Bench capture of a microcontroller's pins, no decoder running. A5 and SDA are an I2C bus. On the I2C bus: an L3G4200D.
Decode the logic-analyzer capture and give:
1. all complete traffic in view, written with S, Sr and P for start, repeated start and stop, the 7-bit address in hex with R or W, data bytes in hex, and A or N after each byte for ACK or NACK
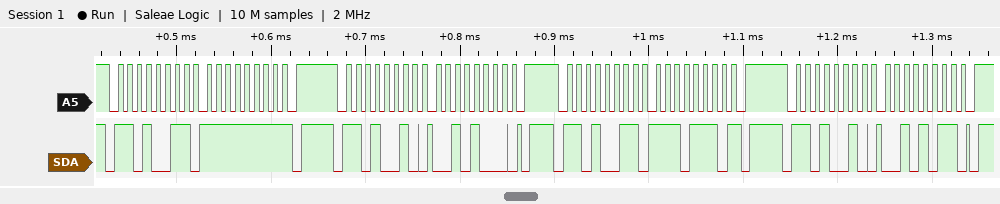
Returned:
S 69R A FF N P S 69W A 28 A P S 69R A EE N P S 69W A 2B A P
